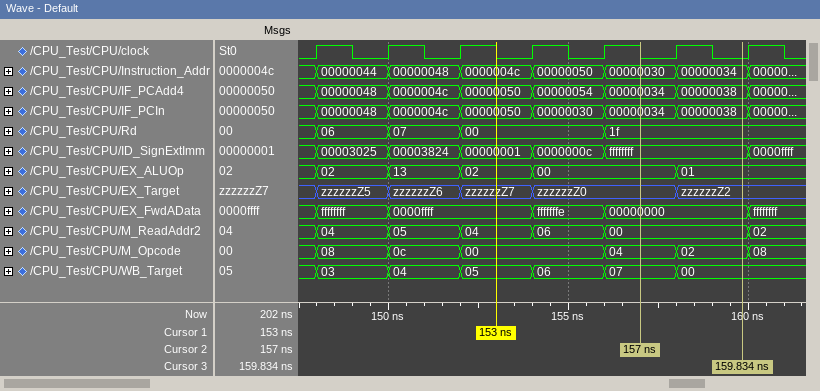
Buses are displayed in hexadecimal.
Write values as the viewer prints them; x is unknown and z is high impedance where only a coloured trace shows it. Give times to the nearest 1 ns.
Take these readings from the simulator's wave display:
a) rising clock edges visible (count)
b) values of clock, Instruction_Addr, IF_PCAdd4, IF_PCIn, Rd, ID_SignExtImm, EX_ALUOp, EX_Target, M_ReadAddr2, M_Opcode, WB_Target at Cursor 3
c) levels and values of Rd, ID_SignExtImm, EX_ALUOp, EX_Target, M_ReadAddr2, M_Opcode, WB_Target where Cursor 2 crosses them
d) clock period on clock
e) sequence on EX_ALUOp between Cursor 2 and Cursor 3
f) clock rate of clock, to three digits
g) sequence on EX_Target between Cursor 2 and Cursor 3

7
clock=0, Instruction_Addr=00000034, IF_PCAdd4=00000038, IF_PCIn=00000038, Rd=1f, ID_SignExtImm=ffffffff, EX_ALUOp=01, EX_Target=zzzzzzZ2, M_ReadAddr2=00, M_Opcode=02, WB_Target=00
Rd=1f, ID_SignExtImm=ffffffff, EX_ALUOp=00, EX_Target=zzzzzzZ0, M_ReadAddr2=00, M_Opcode=04, WB_Target=07
2 ns
00, 01
500 MHz
zzzzzzZ0, zzzzzzZ2
